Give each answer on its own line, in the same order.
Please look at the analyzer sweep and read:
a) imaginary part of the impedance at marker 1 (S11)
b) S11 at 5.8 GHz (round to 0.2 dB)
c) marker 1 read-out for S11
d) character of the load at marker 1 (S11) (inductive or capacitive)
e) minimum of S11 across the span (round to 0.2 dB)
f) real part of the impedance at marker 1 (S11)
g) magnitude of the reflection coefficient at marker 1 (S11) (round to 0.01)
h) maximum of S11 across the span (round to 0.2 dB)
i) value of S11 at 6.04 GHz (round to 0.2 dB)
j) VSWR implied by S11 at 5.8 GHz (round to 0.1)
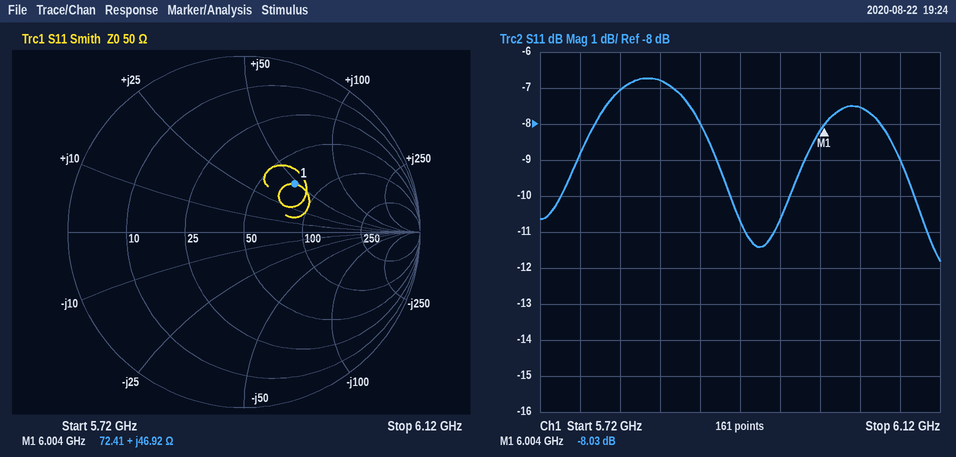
+46.92 Ω
-7.0 dB
-8.03 dB
inductive
-11.8 dB
72.41 Ω
0.40
-6.8 dB
-7.6 dB
2.6
